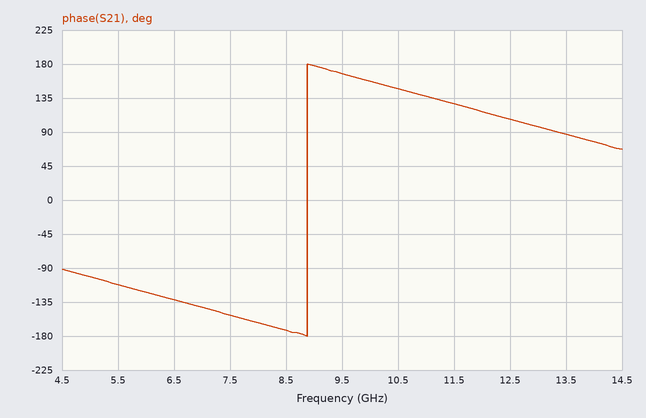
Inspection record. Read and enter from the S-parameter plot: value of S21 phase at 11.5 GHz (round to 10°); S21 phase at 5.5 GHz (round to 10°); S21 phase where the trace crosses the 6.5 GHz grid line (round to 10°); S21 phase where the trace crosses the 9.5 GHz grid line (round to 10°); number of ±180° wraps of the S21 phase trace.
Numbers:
130°
-110°
-130°
170°
1
